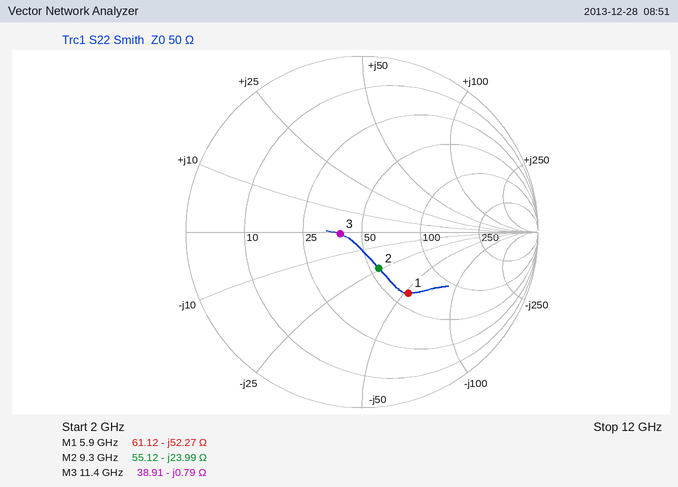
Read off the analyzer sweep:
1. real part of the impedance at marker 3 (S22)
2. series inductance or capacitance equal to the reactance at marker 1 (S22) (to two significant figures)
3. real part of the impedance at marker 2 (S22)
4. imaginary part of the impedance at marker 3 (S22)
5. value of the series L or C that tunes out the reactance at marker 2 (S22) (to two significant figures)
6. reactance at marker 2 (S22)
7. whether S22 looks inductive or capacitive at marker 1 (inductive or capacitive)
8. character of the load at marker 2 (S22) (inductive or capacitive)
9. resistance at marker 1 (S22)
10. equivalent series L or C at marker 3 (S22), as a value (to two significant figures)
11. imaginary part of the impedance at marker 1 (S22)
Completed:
38.91 Ω
520 fF
55.12 Ω
-0.79 Ω
410 pH
-23.99 Ω
capacitive
capacitive
61.12 Ω
18 pF
-52.27 Ω
